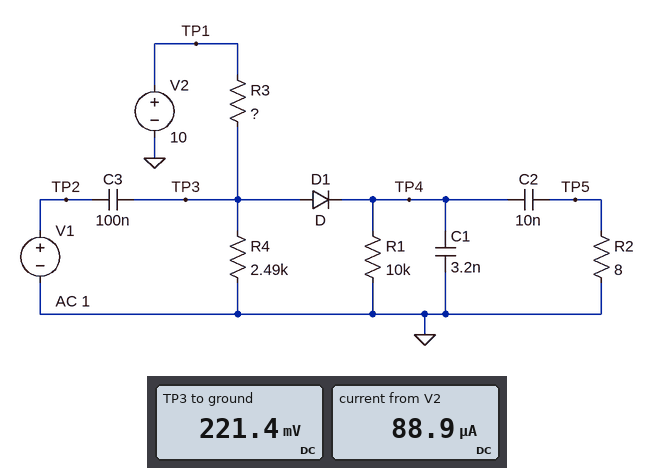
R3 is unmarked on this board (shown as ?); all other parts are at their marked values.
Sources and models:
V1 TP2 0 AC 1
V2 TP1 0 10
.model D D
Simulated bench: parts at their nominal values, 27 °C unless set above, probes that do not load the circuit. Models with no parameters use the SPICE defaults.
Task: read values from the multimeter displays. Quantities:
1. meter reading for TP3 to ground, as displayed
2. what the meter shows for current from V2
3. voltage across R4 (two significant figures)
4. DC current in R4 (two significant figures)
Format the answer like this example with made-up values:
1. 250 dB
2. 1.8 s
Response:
1. 221.4 mV
2. 88.9 µA
3. 220 mV
4. 89 µA
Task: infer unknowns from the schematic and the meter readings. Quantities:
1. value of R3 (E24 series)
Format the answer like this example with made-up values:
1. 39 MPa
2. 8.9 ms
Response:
1. 110 kΩ
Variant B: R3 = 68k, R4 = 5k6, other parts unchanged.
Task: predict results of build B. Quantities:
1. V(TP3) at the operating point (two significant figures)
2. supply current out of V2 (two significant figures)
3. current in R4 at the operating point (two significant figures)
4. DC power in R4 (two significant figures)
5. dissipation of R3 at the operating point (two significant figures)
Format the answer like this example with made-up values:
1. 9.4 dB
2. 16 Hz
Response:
1. 690 mV
2. 140 µA
3. 120 µA
4. 84 µW
5. 1.3 mW
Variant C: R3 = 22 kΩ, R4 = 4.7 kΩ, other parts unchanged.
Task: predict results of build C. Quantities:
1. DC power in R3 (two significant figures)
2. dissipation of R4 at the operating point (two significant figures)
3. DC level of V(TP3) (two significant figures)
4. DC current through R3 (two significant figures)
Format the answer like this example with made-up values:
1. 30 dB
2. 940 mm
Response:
1. 3.3 mW
2. 440 µW
3. 1.4 V
4. 390 µA
